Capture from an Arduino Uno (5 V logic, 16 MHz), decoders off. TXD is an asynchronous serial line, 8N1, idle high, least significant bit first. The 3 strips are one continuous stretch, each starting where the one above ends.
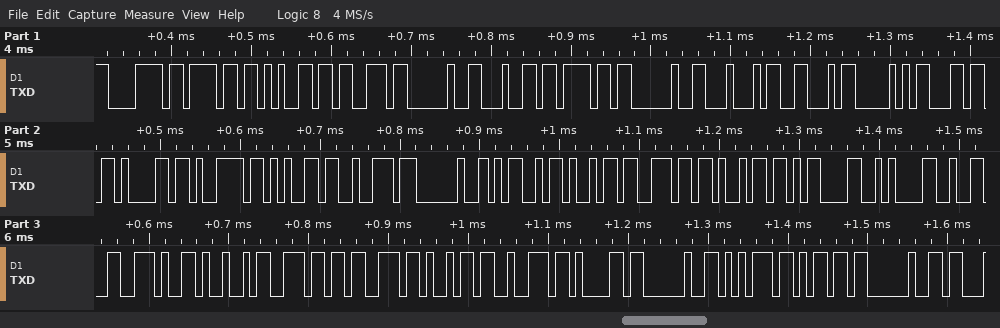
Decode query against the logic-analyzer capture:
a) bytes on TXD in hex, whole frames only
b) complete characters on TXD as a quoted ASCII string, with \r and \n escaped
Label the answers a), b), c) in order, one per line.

a) 78 6F 65 73 20 64 6F 20 44 46 50 6C 61 79 65 72 20 4D 69 6E 69 0D 0A 32 2E 49 6E 73 69 72 61 20 75 6D 20
b) "xoes do DFPlayer Mini\r\n2.Insira um "
